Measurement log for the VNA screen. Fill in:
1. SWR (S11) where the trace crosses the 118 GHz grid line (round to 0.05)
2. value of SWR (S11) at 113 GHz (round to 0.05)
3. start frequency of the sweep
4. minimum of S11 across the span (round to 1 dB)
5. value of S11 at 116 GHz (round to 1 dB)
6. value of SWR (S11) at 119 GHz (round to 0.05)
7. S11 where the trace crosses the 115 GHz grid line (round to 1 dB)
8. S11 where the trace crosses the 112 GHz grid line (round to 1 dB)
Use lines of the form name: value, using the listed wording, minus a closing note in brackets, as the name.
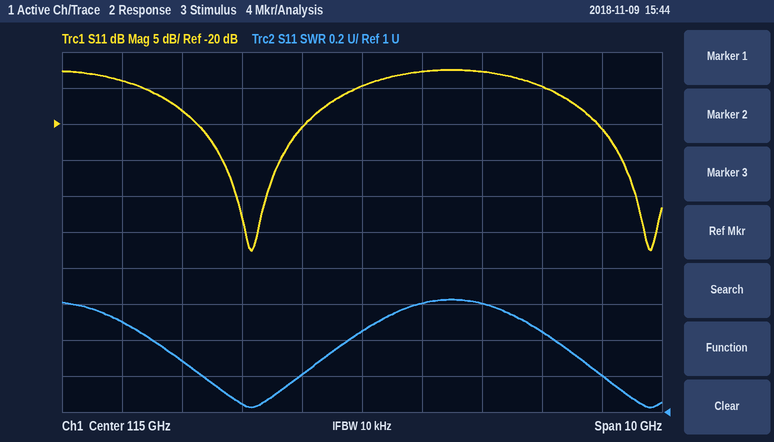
SWR (S11) where the trace crosses the 118 GHz grid line: 1.45
value of SWR (S11) at 113 GHz: 1.05
start frequency of the sweep: 110 GHz
minimum of S11 across the span: -38 dB
value of S11 at 116 GHz: -13 dB
value of SWR (S11) at 119 GHz: 1.20
S11 where the trace crosses the 115 GHz grid line: -15 dB
S11 where the trace crosses the 112 GHz grid line: -18 dB
